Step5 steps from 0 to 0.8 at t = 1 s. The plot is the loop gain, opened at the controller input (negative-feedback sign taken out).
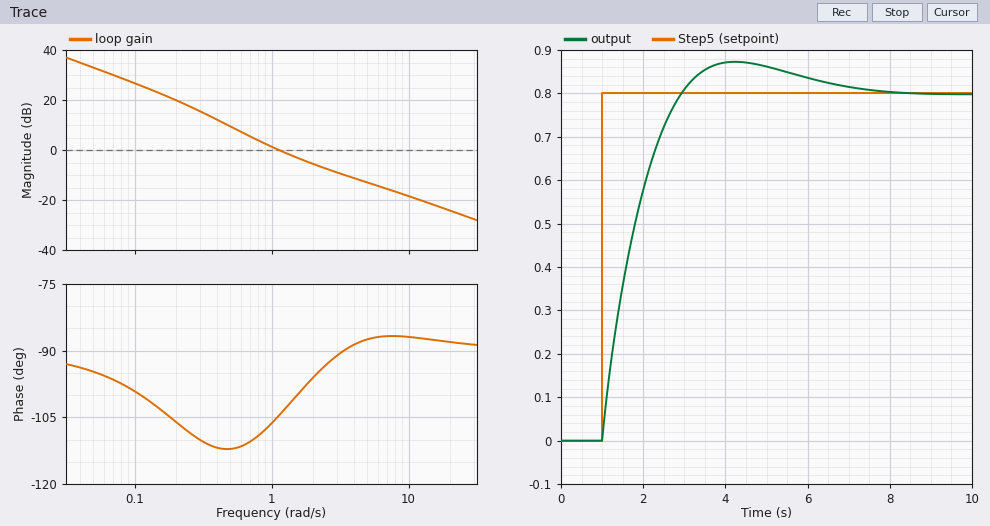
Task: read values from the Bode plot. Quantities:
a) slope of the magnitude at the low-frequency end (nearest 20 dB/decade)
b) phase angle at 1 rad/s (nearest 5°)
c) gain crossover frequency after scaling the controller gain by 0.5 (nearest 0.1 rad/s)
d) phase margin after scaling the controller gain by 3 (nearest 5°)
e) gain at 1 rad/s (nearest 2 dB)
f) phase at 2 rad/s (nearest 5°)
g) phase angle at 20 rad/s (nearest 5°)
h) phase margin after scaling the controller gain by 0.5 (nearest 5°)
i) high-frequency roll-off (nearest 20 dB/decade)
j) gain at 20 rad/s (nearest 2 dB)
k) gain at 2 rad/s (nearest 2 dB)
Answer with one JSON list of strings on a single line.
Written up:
["-20 dB/decade", "-105°", "0.7 rad/s", "90°", "2 dB", "-95°", "-90°", "70°", "-20 dB/decade", "-24 dB", "-6 dB"]
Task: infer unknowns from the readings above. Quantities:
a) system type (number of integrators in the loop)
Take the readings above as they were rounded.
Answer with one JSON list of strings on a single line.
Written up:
["1"]
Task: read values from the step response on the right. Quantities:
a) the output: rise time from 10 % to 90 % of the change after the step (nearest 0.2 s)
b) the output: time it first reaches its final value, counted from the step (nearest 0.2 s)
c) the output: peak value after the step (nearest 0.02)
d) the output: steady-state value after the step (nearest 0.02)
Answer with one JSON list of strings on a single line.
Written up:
["1.4 s", "2.0 s", "0.88", "0.80"]
